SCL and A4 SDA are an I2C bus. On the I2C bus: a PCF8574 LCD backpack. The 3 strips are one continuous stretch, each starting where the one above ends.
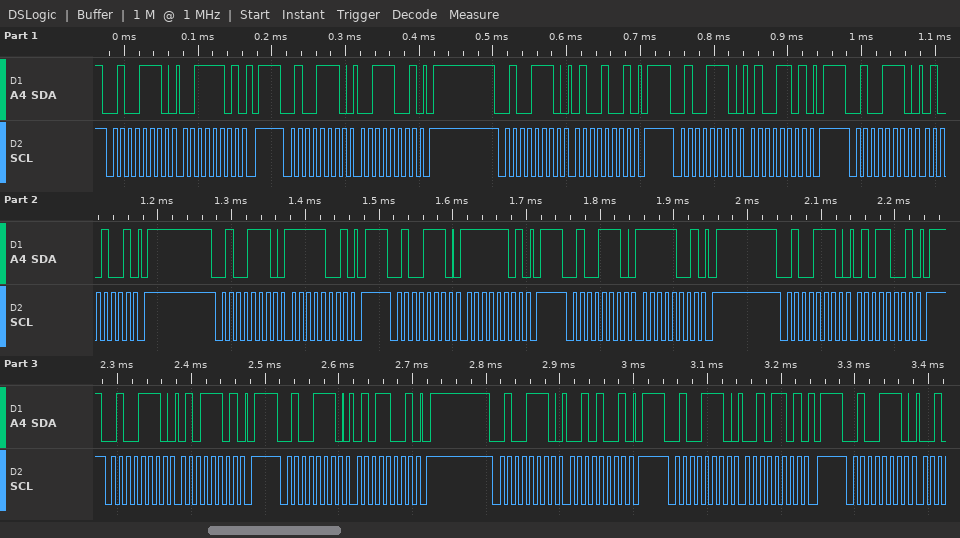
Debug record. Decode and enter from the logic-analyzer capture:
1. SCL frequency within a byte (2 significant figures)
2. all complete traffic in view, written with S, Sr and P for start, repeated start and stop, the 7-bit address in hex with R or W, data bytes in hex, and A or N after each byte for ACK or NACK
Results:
100 kHz
S 27W A 3D A P S 27W A 39 A P S 27W A 49 A P S 27W A 4D A P S 27W A 49 A P S 27W A F9 A P S 27W A FD A P S 27W A F9 A P S 27W A 59 A P S 27W A 5D A P S 27W A 59 A P S 27W A 29 A P S 27W A 2D A P S 27W A
